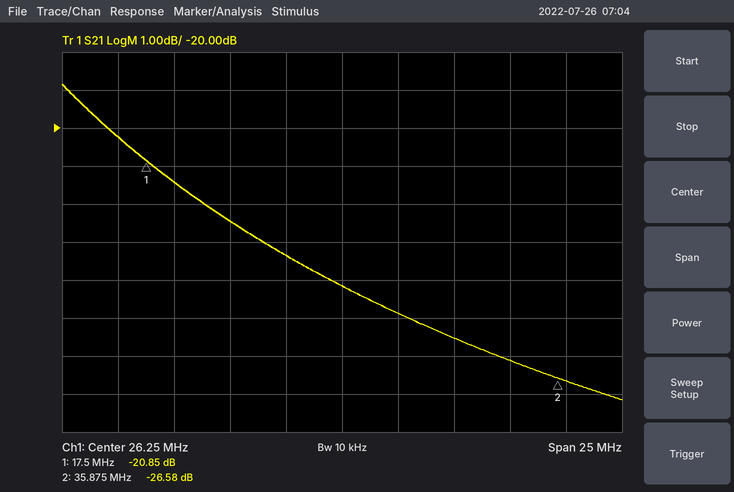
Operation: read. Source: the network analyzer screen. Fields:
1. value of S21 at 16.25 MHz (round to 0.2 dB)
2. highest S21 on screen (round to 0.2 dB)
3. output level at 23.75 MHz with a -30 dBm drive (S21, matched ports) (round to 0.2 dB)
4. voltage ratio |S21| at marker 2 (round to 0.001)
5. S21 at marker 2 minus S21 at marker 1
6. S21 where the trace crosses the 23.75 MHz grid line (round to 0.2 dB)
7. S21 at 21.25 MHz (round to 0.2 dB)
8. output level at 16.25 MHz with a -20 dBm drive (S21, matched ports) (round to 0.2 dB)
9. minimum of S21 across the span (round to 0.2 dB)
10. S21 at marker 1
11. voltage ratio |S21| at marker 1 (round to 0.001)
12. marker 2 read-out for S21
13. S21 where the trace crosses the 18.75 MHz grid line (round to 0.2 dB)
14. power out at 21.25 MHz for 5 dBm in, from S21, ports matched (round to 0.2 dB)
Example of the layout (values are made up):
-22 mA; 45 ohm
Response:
-20.2 dB; -18.8 dB; -53.4 dBm; 0.047; -5.73 dB; -23.4 dB; -22.4 dB; -40.2 dBm; -27.2 dB; -20.85 dB; 0.091; -26.58 dB; -21.4 dB; -17.4 dBm
